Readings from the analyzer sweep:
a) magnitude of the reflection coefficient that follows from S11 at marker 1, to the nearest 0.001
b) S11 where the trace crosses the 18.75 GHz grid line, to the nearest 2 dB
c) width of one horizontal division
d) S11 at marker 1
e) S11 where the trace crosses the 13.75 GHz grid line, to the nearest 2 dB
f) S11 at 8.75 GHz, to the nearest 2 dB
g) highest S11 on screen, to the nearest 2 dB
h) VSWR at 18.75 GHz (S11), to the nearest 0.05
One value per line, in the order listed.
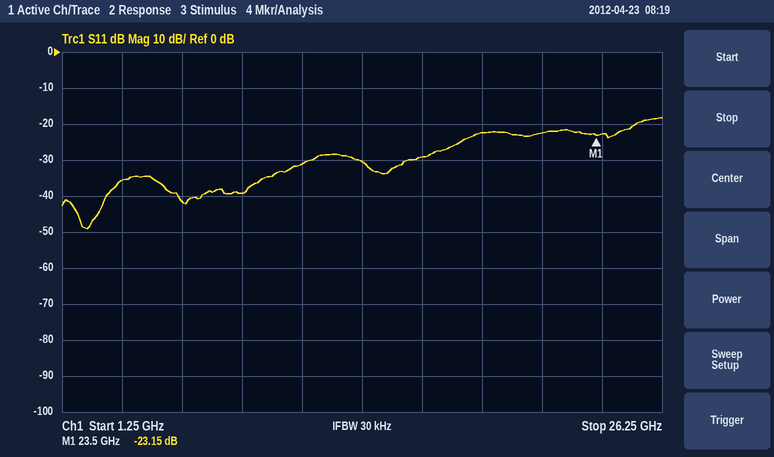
0.070
-22 dB
2.5 GHz
-23.15 dB
-30 dB
-40 dB
-18 dB
1.15
